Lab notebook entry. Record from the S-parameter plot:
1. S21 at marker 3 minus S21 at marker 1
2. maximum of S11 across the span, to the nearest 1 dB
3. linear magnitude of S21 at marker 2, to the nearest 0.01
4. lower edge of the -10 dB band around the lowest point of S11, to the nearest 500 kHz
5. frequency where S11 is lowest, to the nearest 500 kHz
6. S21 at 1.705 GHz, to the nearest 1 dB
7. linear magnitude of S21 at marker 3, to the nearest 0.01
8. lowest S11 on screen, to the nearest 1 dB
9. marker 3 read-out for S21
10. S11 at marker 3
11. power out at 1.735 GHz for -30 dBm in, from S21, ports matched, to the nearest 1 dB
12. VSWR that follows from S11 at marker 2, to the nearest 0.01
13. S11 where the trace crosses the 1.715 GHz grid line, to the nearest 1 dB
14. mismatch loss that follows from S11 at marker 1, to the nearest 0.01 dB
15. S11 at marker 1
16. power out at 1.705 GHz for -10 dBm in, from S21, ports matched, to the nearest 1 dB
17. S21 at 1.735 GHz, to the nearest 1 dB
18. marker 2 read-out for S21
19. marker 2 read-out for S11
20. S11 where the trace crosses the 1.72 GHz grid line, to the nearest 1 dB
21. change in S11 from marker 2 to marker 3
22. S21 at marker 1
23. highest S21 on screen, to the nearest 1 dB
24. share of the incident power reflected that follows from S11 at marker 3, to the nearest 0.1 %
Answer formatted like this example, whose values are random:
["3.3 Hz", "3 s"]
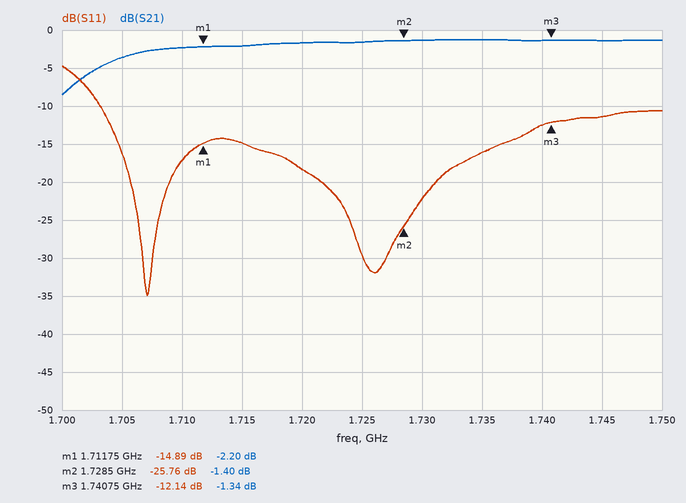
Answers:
["0.86 dB", "-5 dB", "0.85", "1.7030 GHz", "1.7070 GHz", "-4 dB", "0.86", "-35 dB", "-1.34 dB", "-12.14 dB", "-31 dBm", "1.11", "-15 dB", "0.14 dB", "-14.89 dB", "-14 dBm", "-1 dB", "-1.40 dB", "-25.76 dB", "-18 dB", "13.62 dB", "-2.20 dB", "-1 dB", "6.1 %"]
